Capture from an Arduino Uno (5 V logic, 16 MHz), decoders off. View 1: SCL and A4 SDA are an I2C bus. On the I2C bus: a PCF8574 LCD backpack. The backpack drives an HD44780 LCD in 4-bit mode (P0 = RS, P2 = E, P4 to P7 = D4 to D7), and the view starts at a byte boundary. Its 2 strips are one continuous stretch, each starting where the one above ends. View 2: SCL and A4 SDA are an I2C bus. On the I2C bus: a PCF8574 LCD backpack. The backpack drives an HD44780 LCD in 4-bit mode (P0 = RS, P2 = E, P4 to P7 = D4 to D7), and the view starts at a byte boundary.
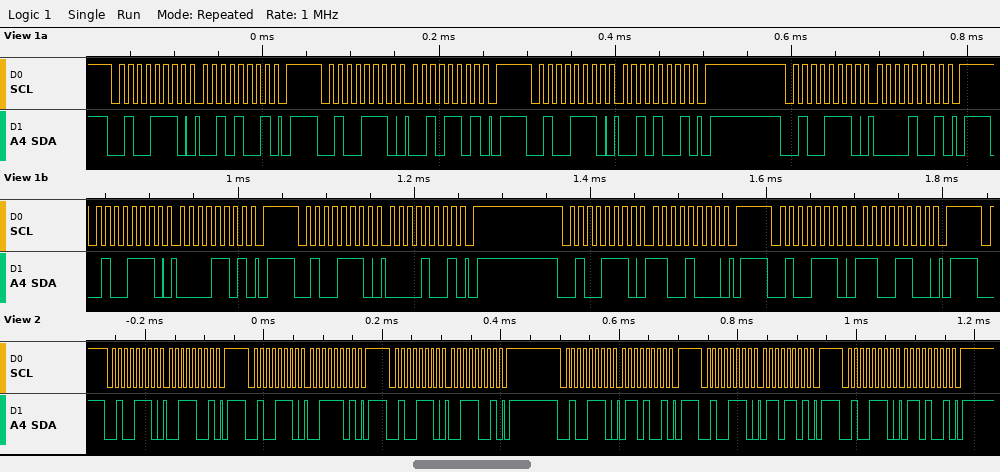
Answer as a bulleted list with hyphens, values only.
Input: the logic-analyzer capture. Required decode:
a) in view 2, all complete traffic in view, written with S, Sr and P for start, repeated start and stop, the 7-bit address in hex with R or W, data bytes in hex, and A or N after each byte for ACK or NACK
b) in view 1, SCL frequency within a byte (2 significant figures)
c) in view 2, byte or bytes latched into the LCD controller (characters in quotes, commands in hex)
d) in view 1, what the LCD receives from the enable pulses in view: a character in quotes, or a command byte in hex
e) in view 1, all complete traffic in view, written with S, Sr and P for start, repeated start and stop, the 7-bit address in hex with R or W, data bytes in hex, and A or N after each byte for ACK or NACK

- S 27W A 39 A P S 27W A 3D A P S 27W A 39 A P S 27W A 69 A P S 27W A 6D A P S 27W A 69 A P
- 100 kHz
- '6'
- ' '
- S 27W A 29 A P S 27W A 2D A P S 27W A 29 A P S 27W A 09 A P S 27W A 0D A P S 27W A 09 A P S 27W A C8 A P S 27W A CC A P
